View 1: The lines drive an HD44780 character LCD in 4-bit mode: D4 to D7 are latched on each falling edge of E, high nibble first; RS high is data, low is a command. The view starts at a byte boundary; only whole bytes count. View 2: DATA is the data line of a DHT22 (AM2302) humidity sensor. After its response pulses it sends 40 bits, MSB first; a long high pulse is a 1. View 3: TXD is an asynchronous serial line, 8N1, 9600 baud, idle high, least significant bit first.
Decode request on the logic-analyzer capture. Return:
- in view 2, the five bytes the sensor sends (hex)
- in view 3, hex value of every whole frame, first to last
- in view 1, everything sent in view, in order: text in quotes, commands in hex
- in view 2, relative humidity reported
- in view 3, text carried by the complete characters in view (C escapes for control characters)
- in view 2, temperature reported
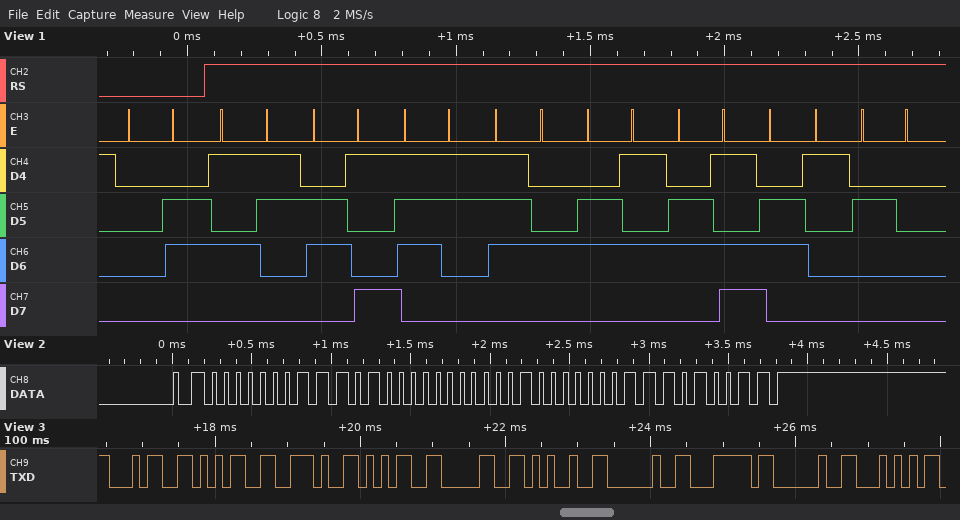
01 D0 01 01 D3
34 35 2E 35 30 25 20 7C 20 54
0x06 "Sistema "
46.4 %
"45.50% | T"
25.7 °C
